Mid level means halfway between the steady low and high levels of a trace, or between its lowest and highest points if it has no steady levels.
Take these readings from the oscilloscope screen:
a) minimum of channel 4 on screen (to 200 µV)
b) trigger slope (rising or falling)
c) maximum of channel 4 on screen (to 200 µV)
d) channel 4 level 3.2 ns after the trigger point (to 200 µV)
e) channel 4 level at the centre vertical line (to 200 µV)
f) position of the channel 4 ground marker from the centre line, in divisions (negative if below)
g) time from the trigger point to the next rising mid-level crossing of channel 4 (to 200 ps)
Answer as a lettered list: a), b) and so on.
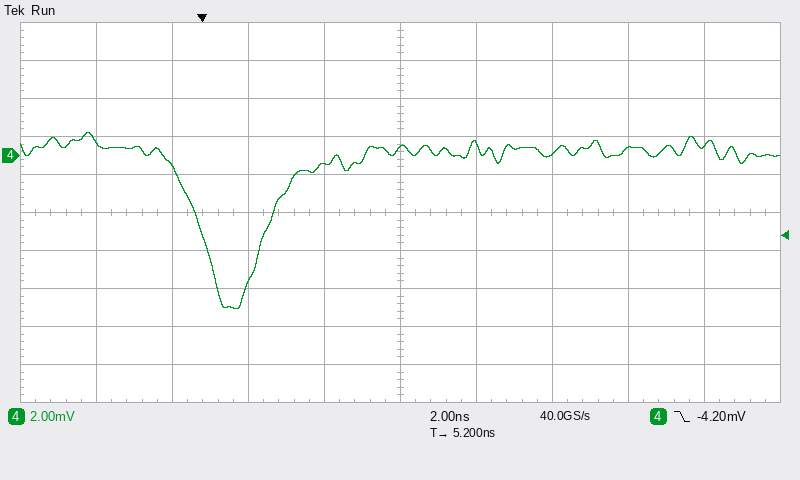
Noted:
a) -8.0 mV
b) falling
c) 1.2 mV
d) -400 µV
e) 400 µV
f) +1.5 div
g) 1.8 ns
